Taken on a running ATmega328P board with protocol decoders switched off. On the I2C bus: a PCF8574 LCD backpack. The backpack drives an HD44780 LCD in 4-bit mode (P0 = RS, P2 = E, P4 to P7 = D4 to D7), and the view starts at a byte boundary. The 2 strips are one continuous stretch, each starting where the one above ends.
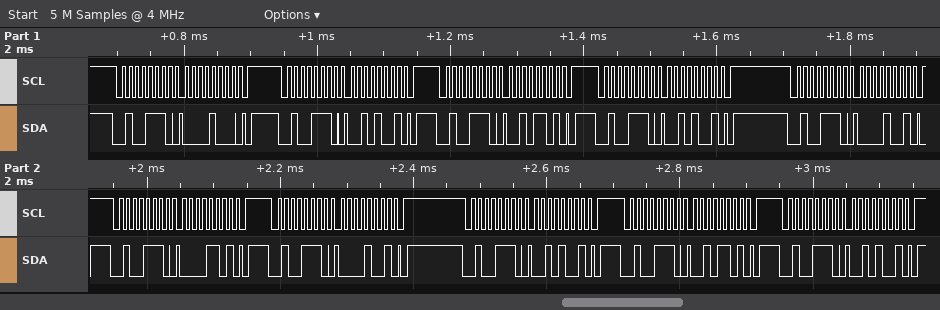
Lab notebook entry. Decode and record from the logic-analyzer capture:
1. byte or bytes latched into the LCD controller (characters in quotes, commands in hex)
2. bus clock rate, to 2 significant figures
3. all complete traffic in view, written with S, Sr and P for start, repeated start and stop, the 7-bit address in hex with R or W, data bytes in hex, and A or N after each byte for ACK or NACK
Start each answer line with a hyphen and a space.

- ' '
- 100 kHz
- S 27W A 08 A P S 27W A 29 A P S 27W A 2D A P S 27W A 29 A P S 27W A 09 A P S 27W A 0D A P S 27W A 09 A P S 27W A 29 A P S 27W A 2D A P S 27W A 29 A P
